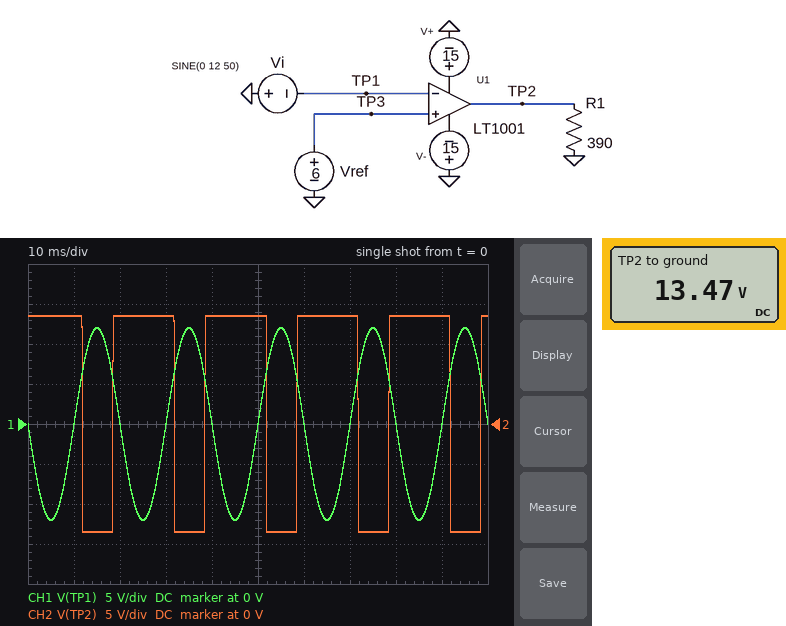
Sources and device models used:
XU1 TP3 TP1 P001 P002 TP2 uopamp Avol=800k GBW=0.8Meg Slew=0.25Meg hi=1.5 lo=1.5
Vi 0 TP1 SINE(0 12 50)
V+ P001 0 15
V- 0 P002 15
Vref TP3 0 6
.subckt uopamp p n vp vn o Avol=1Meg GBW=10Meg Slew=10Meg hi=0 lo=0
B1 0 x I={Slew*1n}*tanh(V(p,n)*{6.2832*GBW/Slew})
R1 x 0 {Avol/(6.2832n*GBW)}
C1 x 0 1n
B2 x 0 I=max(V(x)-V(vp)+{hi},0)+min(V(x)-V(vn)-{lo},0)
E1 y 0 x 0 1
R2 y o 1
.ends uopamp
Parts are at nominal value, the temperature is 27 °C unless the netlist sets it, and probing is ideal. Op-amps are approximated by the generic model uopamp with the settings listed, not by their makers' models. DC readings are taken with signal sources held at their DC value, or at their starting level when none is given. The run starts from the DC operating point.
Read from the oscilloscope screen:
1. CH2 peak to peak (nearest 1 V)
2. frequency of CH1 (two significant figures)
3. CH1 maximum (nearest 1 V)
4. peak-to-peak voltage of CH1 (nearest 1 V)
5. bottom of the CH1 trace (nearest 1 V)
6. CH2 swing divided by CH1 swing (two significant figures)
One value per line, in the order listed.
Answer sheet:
27 V
50 Hz
12 V
24 V
-12 V
1.1
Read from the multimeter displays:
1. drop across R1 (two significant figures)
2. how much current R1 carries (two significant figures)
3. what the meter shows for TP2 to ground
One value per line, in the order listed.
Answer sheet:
13 V
35 mA
13.47 V
